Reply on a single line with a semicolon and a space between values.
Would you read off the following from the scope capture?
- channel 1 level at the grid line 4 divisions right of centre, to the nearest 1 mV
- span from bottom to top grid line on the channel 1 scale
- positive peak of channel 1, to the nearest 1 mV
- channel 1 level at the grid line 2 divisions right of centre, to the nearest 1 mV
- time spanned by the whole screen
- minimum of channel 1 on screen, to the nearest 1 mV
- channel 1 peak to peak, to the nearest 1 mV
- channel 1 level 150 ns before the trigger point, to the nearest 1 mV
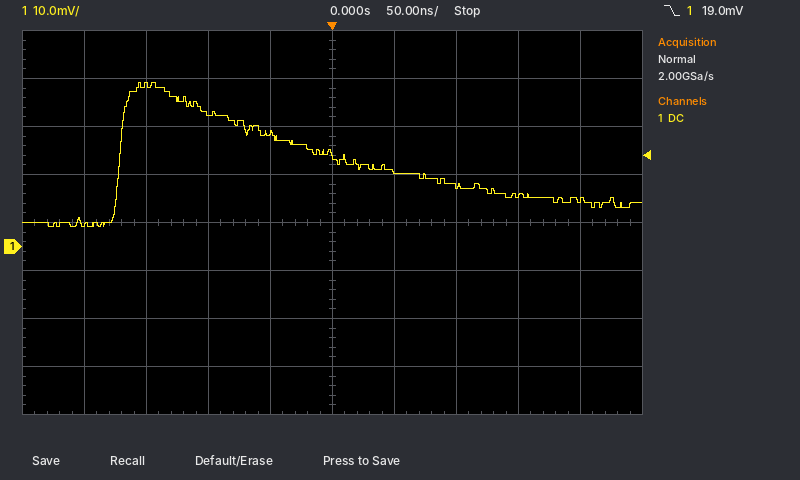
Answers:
10 mV; 80 mV; 34 mV; 13 mV; 500 ns; 4 mV; 30 mV; 34 mV
